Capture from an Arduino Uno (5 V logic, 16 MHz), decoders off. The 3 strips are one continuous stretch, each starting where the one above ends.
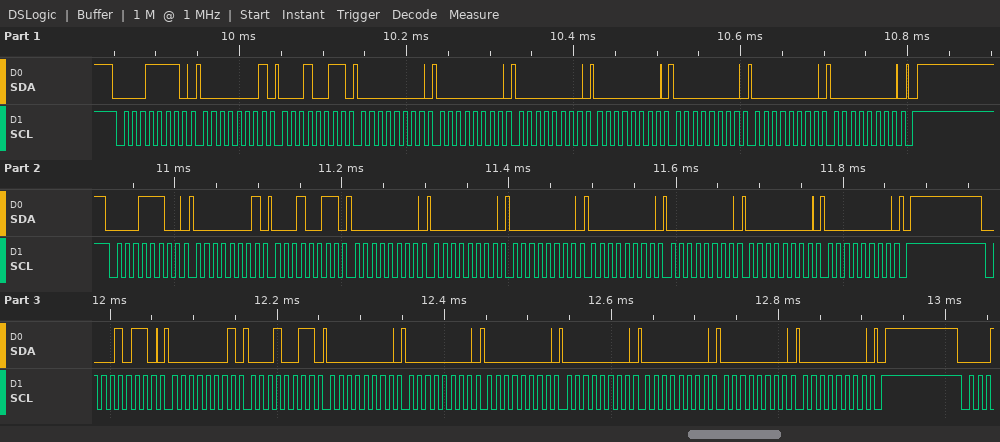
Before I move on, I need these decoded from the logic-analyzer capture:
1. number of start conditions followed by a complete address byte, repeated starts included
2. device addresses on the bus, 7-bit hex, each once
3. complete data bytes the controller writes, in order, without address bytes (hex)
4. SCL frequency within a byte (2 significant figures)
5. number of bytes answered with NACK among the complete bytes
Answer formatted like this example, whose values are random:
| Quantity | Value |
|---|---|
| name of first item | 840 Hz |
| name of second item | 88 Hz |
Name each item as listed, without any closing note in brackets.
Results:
| Quantity | Value |
|---|---|
| number of start conditions followed by a complete address byte, repeated starts included | 3 |
| device addresses on the bus, 7-bit hex, each once | 0x0F 0x0E 0x0B |
| complete data bytes the controller writes, in order, without address bytes | 01 13 00 00 00 00 00 00 00 01 13 00 00 00 00 00 00 00 01 13 00 00 00 00 00 00 00 |
| SCL frequency within a byte | 100 kHz |
| number of bytes answered with NACK among the complete bytes | 0 |
